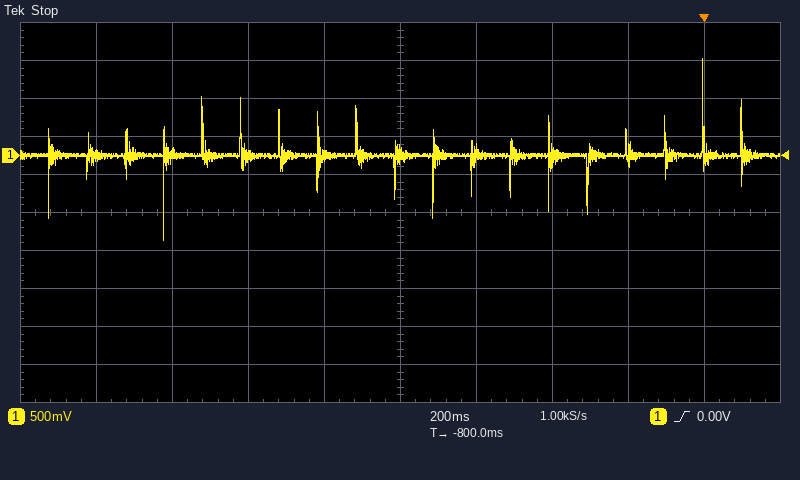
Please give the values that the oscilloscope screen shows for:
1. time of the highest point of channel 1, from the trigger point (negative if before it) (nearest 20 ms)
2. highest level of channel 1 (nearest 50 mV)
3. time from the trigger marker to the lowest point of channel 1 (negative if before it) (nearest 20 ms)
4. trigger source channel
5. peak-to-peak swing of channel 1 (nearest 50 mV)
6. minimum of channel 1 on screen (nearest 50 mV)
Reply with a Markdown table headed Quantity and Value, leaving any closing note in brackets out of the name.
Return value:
| Quantity | Value |
|---|---|
| time of the highest point of channel 1, from the trigger point (negative if before it) | 0 ms |
| highest level of channel 1 | 1.30 V |
| time from the trigger marker to the lowest point of channel 1 (negative if before it) | -1.42 s |
| trigger source channel | channel 1 |
| peak-to-peak swing of channel 1 | 2.40 V |
| minimum of channel 1 on screen | -1.10 V |
